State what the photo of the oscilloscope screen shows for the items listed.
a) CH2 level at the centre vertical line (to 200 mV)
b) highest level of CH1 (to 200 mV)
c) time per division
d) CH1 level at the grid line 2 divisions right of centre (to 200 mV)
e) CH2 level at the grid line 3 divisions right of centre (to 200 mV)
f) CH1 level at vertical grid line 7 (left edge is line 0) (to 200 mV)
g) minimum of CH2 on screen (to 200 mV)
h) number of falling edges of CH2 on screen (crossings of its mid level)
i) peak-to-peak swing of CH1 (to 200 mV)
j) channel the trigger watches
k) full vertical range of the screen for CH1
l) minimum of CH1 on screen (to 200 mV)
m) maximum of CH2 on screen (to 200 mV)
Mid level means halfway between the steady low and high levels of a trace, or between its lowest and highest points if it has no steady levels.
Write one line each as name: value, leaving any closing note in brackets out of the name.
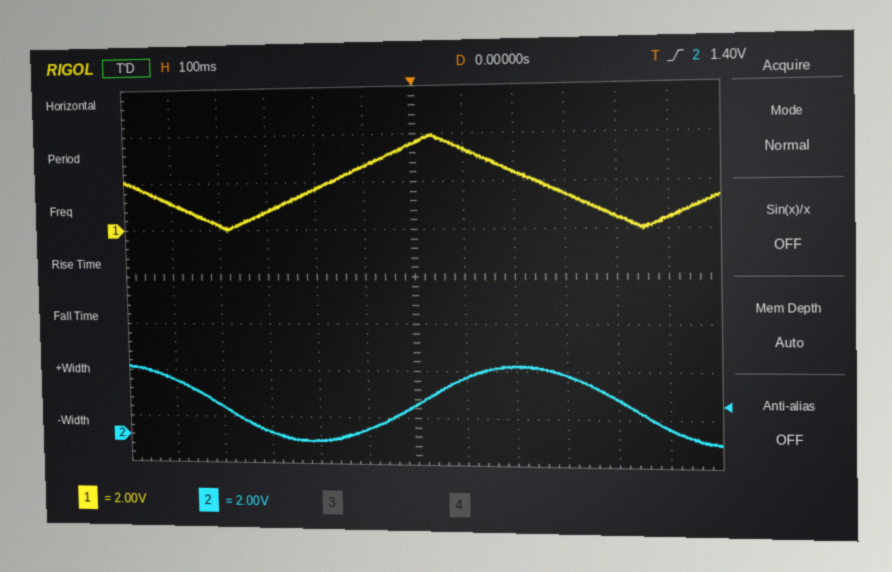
CH2 level at the centre vertical line: 1.4 V
highest level of CH1: 4.0 V
time per division: 100 ms
CH1 level at the grid line 2 divisions right of centre: 2.4 V
CH2 level at the grid line 3 divisions right of centre: 2.6 V
CH1 level at vertical grid line 7 (left edge is line 0): 3.4 V
minimum of CH2 on screen: -200 mV
number of falling edges of CH2 on screen: 2
peak-to-peak swing of CH1: 4.0 V
channel the trigger watches: CH2
full vertical range of the screen for CH1: 16 V
minimum of CH1 on screen: 0.0 V
maximum of CH2 on screen: 3.0 V
